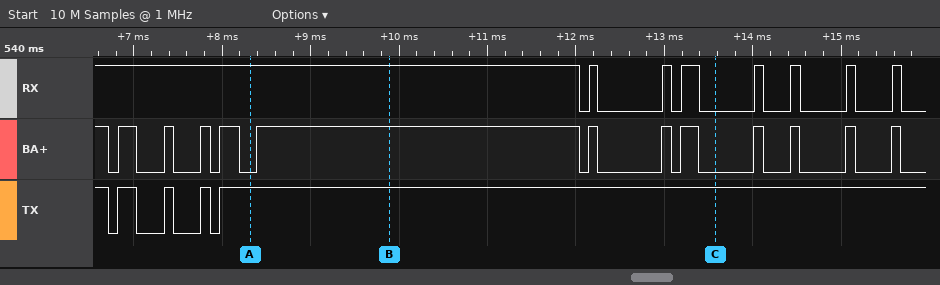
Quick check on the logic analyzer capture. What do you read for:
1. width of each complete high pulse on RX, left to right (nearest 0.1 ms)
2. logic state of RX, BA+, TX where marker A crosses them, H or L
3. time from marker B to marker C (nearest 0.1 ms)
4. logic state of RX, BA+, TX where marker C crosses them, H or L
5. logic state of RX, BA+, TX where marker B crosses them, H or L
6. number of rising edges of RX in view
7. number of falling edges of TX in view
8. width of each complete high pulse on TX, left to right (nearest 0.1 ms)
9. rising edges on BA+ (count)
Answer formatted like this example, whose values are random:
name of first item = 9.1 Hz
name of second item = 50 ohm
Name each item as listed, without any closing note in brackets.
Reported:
width of each complete high pulse on RX, left to right = 0.1 ms, 0.1 ms, 0.2 ms, 0.1 ms, 0.1 ms, 0.1 ms, 0.1 ms
logic state of RX, BA+, TX where marker A crosses them, H or L = RX=H, BA+=L, TX=H
time from marker B to marker C = 3.7 ms
logic state of RX, BA+, TX where marker C crosses them, H or L = RX=L, BA+=L, TX=H
logic state of RX, BA+, TX where marker B crosses them, H or L = RX=H, BA+=H, TX=H
number of rising edges of RX in view = 7
number of falling edges of TX in view = 4
width of each complete high pulse on TX, left to right = 0.2 ms, 0.1 ms, 0.1 ms
rising edges on BA+ = 12
